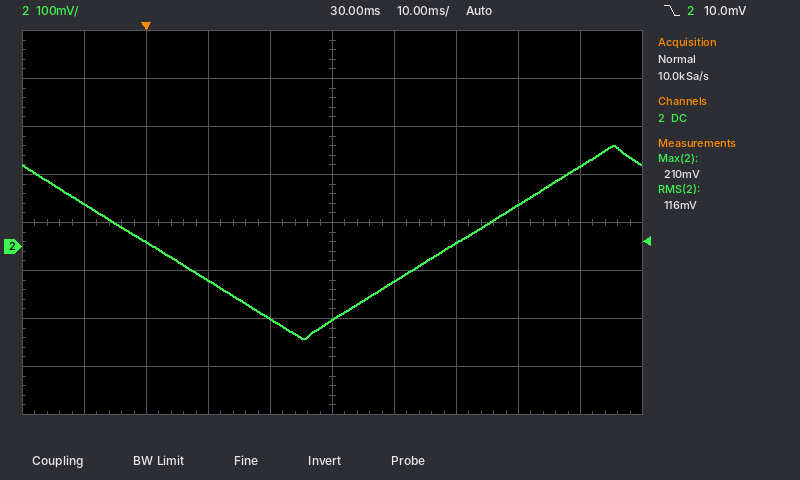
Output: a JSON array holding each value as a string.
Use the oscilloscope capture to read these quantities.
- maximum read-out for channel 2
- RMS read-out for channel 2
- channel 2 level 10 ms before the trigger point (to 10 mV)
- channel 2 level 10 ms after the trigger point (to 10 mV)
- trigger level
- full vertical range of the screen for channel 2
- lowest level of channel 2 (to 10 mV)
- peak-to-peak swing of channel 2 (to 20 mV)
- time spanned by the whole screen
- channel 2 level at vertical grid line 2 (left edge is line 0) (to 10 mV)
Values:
["210 mV", "116 mV", "90 mV", "-70 mV", "10.0 mV", "800 mV", "-190 mV", "400 mV", "100 ms", "10 mV"]
